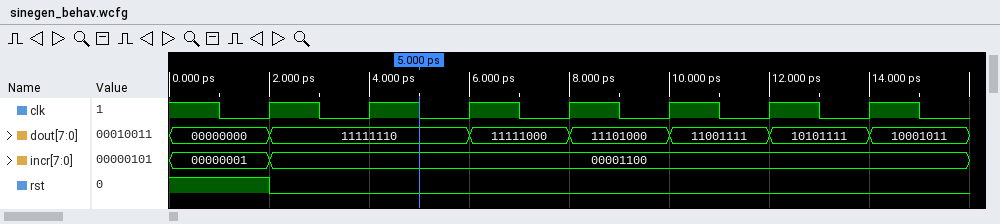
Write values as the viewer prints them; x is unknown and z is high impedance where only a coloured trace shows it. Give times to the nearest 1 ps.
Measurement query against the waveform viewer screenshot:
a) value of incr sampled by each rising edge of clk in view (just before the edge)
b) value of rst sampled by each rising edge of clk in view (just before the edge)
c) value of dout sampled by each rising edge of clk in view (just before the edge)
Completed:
00000001, 00001100, 00001100, 00001100, 00001100, 00001100, 00001100
1 0 0 0 0 0 0
00000000, 11111110, 11111110, 11111000, 11101000, 11001111, 10101111
